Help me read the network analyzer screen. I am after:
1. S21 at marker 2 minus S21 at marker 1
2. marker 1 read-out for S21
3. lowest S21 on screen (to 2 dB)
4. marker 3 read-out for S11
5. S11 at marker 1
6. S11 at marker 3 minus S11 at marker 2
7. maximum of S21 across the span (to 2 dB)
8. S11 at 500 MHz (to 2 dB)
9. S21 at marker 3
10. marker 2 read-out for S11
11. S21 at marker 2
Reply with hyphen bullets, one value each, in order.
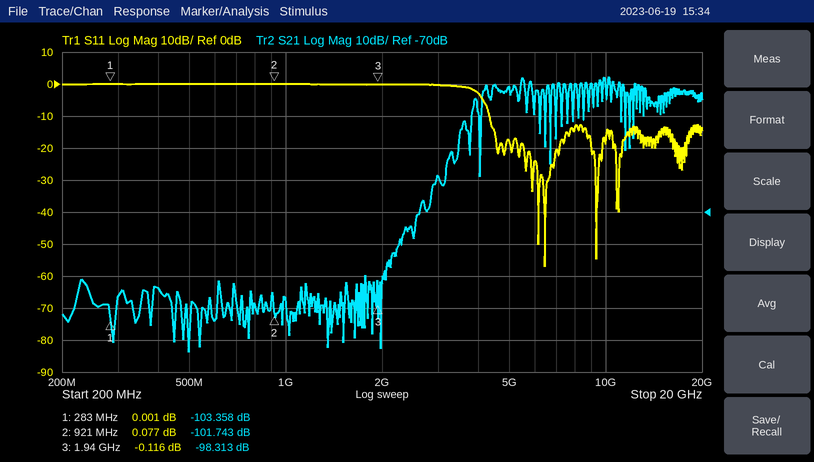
- 1.615 dB
- -103.358 dB
- -114 dB
- -0.116 dB
- 0.001 dB
- -0.193 dB
- -28 dB
- 0 dB
- -98.313 dB
- 0.077 dB
- -101.743 dB
